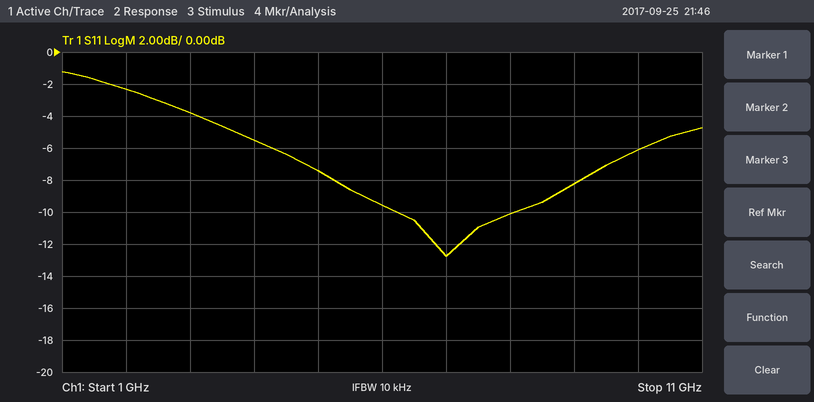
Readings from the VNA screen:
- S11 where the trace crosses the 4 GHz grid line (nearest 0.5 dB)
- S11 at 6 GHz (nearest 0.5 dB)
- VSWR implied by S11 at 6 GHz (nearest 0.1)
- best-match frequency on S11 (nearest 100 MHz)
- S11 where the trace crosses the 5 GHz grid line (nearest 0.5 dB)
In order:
-5.5 dB
-9.5 dB
2.0
7.0 GHz
-7.5 dB
